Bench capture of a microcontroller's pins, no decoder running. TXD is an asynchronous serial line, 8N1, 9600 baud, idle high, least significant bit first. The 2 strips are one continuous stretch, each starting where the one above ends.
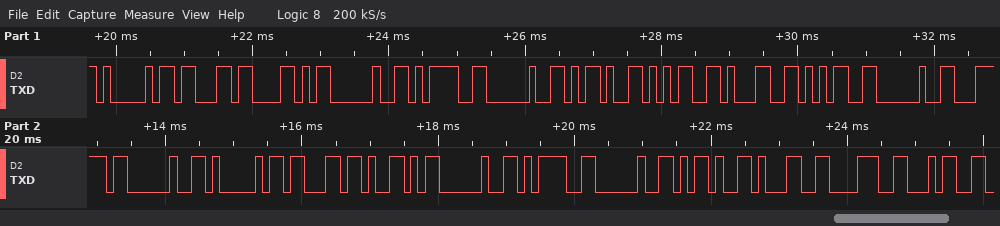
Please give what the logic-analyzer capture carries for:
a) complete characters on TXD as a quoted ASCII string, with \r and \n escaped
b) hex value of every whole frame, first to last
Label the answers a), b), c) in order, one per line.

a) "AcX = -515 | AcY = -184"
b) 41 63 58 20 3D 20 2D 35 31 35 20 7C 20 41 63 59 20 3D 20 2D 31 38 34
